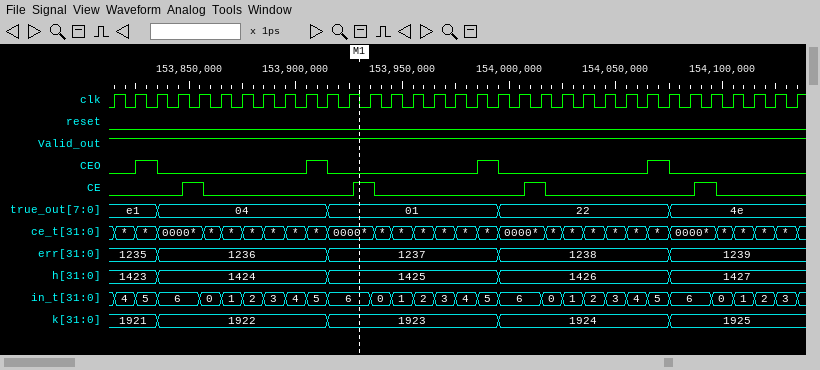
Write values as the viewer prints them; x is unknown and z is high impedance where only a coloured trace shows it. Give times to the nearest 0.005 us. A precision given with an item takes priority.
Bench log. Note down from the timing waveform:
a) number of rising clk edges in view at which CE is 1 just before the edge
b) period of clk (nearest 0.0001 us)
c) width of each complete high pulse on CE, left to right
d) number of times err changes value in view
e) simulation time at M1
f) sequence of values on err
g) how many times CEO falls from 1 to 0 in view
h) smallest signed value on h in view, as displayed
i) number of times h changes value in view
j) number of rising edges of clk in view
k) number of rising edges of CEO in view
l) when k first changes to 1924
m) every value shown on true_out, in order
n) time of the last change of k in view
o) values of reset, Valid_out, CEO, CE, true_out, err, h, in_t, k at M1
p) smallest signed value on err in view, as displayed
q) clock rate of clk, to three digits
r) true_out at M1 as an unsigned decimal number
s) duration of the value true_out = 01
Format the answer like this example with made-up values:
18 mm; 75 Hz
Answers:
4; 0.01 us; 0.01 us, 0.01 us, 0.01 us, 0.01 us; 4; 153.93 us; 1235, 1236, 1237, 1238, 1239; 4; 1423; 4; 33; 4; 153.995 us; e1, 04, 01, 22, 4e; 154.075 us; reset=0, Valid_out=1, CEO=0, CE=1, true_out=01, err=1237, h=1425, in_t=6, k=1923; 1235; 100 MHz; 1; 0.08 us
